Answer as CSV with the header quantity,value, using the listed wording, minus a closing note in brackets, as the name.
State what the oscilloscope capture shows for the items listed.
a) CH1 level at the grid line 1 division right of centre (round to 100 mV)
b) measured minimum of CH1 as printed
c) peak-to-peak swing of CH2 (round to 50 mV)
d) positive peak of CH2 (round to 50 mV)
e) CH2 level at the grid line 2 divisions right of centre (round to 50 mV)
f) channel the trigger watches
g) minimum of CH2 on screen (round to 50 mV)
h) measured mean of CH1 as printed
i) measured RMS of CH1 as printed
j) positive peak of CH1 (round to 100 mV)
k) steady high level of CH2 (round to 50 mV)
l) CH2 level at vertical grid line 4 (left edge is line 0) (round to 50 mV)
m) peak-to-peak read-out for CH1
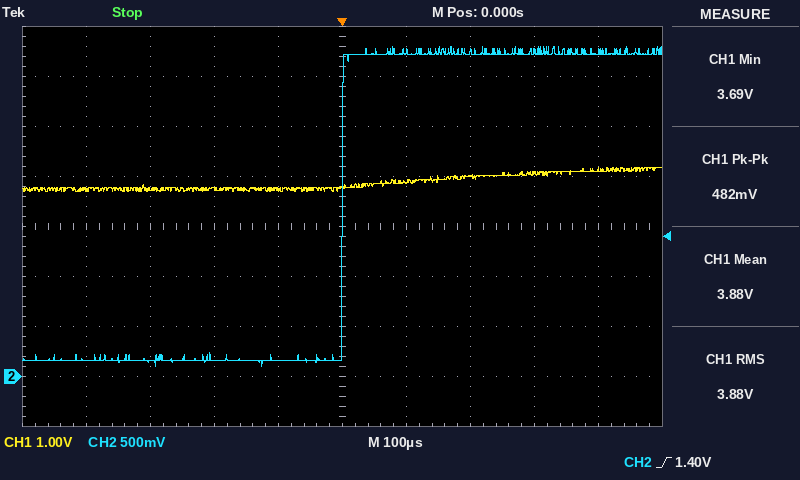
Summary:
quantity,value
CH1 level at the grid line 1 division right of centre,3.9 V
measured minimum of CH1 as printed,3.69 V
peak-to-peak swing of CH2,3.20 V
positive peak of CH2,3.30 V
CH2 level at the grid line 2 divisions right of centre,3.25 V
channel the trigger watches,CH2
minimum of CH2 on screen,100 mV
measured mean of CH1 as printed,3.88 V
measured RMS of CH1 as printed,3.88 V
positive peak of CH1,4.2 V
steady high level of CH2,3.20 V
CH2 level at vertical grid line 4 (left edge is line 0),150 mV
peak-to-peak read-out for CH1,482 mV
